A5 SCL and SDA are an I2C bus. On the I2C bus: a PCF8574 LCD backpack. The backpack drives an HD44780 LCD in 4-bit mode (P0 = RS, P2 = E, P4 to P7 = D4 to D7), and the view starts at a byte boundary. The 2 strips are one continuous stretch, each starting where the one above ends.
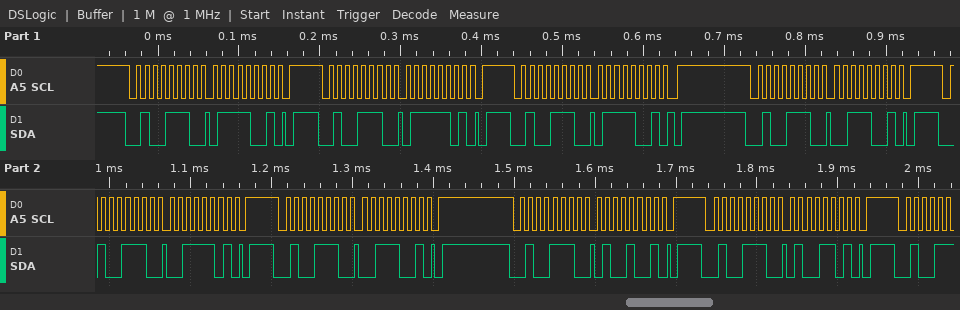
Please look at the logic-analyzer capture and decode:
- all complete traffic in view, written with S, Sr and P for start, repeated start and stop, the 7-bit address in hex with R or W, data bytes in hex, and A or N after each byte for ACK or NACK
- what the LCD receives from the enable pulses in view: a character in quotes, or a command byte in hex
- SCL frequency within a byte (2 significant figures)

S 27W A 79 A P S 27W A 7D A P S 27W A 79 A P S 27W A 39 A P S 27W A 3D A P S 27W A 39 A P S 27W A 49 A P S 27W A 4D A P
's'
100 kHz
